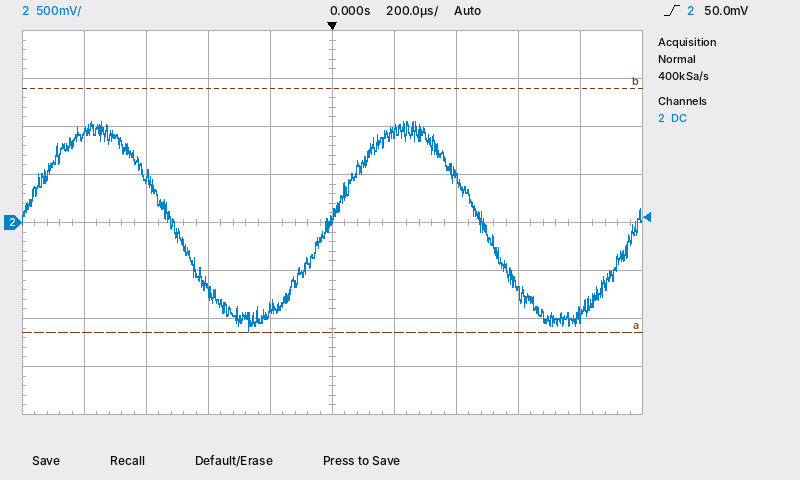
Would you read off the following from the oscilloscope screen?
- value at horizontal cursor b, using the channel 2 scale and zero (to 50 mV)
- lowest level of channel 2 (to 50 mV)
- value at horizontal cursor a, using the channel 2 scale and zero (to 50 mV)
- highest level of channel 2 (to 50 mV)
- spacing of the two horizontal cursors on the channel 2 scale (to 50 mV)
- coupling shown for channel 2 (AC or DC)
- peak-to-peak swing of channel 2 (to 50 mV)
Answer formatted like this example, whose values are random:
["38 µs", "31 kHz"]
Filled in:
["1.40 V", "-1.15 V", "-1.15 V", "1.05 V", "2.55 V", "DC", "2.20 V"]
